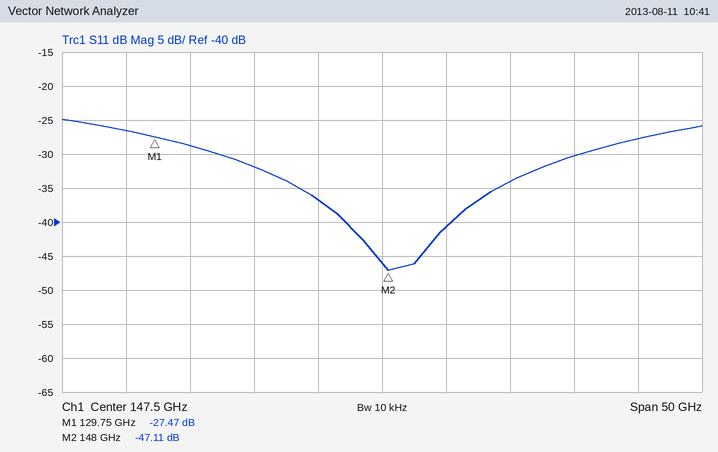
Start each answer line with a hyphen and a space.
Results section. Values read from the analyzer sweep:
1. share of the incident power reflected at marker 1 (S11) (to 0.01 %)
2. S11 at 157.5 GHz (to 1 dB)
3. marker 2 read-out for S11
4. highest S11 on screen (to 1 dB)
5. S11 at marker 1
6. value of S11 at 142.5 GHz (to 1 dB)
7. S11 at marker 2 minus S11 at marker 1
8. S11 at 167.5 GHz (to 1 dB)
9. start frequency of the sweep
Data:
- 0.18 %
- -34 dB
- -47.11 dB
- -25 dB
- -27.47 dB
- -37 dB
- -19.64 dB
- -28 dB
- 122.5 GHz
